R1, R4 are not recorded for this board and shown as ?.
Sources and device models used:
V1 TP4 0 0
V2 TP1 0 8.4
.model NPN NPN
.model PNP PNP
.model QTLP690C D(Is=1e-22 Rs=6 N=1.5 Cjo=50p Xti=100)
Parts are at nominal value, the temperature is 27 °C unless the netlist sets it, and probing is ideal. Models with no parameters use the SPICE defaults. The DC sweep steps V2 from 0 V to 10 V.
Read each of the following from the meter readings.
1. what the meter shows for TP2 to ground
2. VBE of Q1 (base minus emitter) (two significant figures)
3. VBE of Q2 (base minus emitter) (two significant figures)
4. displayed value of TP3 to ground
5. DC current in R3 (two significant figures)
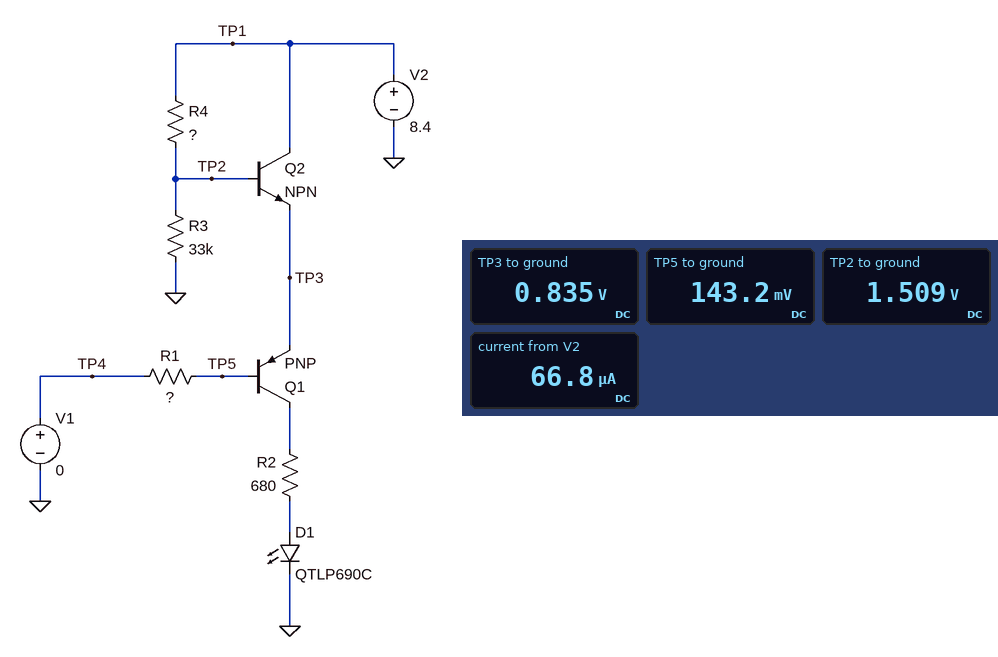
1.509 V
-690 mV
670 mV
0.835 V
46 µA
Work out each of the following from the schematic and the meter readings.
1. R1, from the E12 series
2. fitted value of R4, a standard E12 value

6.8 kΩ
150 kΩ
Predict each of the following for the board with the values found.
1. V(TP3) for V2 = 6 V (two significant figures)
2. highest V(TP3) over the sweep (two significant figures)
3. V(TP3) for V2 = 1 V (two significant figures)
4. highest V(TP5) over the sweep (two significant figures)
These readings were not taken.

550 mV
1.1 V
90 mV
370 mV
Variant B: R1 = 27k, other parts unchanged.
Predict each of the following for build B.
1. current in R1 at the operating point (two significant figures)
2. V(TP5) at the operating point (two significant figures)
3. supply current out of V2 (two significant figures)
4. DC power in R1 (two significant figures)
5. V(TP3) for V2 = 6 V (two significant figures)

7.4 µA
200 mV
53 µA
1.5 µW
550 mV
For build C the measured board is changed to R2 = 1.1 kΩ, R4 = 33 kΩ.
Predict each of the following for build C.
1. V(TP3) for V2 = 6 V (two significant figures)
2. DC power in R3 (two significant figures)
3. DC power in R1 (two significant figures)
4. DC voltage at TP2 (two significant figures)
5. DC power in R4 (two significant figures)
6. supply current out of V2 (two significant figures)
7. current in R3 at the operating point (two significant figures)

2.1 V
470 µW
820 µW
3.9 V
600 µW
1.7 mA
120 µA
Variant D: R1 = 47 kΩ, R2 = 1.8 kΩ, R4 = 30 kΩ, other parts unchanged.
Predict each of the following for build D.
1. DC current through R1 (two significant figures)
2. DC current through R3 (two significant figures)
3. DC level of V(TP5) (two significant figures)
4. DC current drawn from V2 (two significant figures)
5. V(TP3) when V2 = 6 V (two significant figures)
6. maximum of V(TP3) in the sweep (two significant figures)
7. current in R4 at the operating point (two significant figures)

57 µA
130 µA
2.7 V
1.1 mA
2.3 V
4.2 V
140 µA
